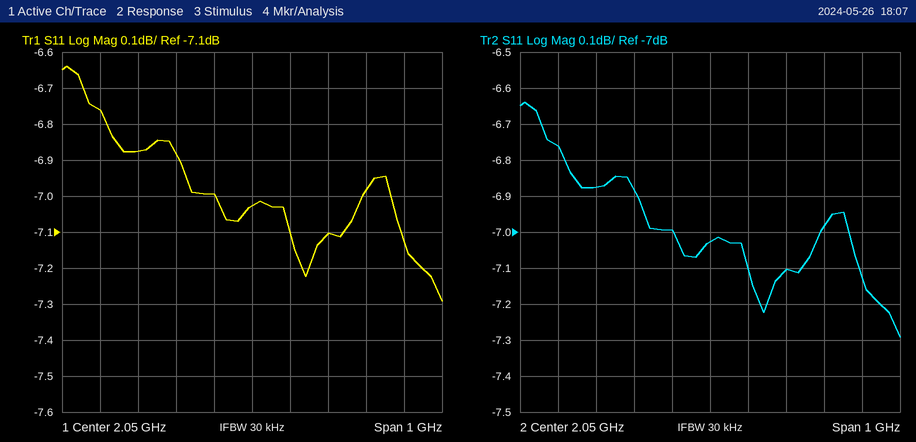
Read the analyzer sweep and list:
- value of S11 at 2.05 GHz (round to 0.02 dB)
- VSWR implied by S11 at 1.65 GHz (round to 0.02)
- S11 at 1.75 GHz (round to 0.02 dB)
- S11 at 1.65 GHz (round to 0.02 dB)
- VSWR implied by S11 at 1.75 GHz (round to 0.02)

-7.02 dB
2.70
-6.88 dB
-6.76 dB
2.66
